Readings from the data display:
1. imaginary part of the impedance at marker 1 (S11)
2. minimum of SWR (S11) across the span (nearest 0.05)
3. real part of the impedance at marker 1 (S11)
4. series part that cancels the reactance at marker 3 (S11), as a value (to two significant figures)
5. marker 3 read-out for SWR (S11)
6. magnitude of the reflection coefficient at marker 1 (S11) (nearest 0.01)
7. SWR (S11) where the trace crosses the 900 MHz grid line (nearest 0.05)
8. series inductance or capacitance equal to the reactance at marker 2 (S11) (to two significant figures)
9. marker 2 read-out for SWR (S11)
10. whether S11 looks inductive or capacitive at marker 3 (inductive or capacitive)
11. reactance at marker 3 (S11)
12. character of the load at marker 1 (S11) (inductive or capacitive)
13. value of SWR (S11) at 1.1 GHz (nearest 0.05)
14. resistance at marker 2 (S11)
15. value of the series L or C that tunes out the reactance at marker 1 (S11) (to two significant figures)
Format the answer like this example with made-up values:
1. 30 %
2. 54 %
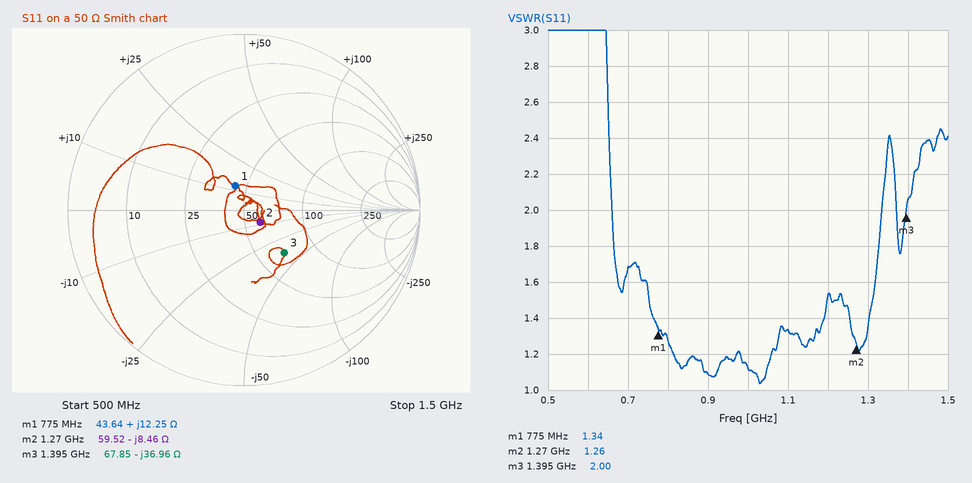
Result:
1. +12.25 Ω
2. 1.05
3. 43.64 Ω
4. 4.2 nH
5. 2.00
6. 0.15
7. 1.10
8. 15 pF
9. 1.26
10. capacitive
11. -36.96 Ω
12. inductive
13. 1.35
14. 59.52 Ω
15. 17 pF
